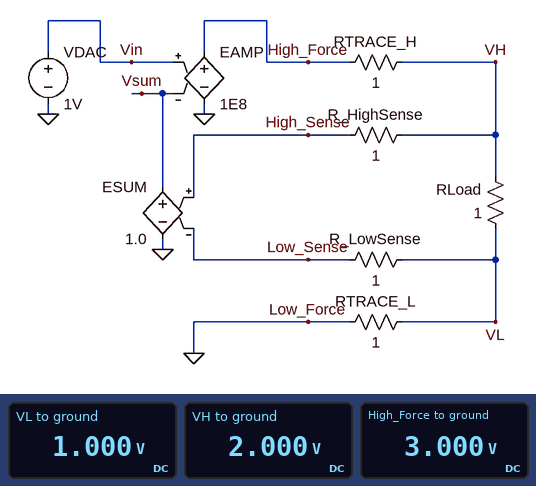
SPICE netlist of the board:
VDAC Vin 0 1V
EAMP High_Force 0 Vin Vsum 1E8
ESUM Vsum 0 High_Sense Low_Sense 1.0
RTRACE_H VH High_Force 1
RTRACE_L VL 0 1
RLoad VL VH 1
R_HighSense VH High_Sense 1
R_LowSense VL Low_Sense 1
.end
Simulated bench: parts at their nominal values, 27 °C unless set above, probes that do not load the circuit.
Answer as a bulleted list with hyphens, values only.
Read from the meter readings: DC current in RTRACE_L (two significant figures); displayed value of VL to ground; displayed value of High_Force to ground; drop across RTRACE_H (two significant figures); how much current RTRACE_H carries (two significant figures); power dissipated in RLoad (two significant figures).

- 1.0 A
- 1.000 V
- 3.000 V
- 1.0 V
- 1.0 A
- 1.0 W
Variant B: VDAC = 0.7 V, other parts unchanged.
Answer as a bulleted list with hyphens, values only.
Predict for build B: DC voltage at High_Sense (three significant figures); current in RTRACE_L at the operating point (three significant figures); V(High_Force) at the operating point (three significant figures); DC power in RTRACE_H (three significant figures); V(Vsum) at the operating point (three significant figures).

- 1.40 V
- 700 mA
- 2.10 V
- 490 mW
- 700 mV
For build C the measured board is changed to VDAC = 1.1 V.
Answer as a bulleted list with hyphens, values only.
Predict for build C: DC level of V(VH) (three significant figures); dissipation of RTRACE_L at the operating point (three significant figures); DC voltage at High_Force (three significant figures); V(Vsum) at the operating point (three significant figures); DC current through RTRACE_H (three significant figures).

- 2.20 V
- 1.21 W
- 3.30 V
- 1.10 V
- 1.10 A
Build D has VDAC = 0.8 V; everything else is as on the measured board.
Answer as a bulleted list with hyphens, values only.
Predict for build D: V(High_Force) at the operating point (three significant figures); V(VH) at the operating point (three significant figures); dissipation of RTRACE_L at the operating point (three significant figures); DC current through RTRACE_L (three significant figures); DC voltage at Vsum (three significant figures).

- 2.40 V
- 1.60 V
- 640 mW
- 800 mA
- 800 mV
